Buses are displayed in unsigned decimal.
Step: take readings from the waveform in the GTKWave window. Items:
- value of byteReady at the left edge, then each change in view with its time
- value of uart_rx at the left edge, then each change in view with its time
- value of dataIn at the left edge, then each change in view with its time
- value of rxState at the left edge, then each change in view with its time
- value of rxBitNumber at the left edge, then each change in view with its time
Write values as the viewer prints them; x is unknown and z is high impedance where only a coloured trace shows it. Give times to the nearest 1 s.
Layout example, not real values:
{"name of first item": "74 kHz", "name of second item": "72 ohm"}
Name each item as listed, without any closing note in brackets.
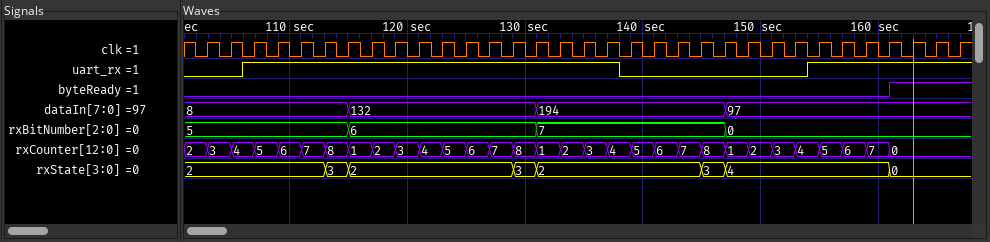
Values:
{"value of byteReady at the left edge, then each change in view with its time": "0, 1 at 161 s", "value of uart_rx at the left edge, then each change in view with its time": "0, 1 at 106 s, 0 at 138 s, 1 at 154 s", "value of dataIn at the left edge, then each change in view with its time": "8, 132 at 115 s, 194 at 131 s, 97 at 147 s", "value of rxState at the left edge, then each change in view with its time": "2, 3 at 113 s, 2 at 115 s, 3 at 129 s, 2 at 131 s, 3 at 145 s, 4 at 147 s, 0 at 161 s", "value of rxBitNumber at the left edge, then each change in view with its time": "5, 6 at 115 s, 7 at 131 s, 0 at 147 s"}
